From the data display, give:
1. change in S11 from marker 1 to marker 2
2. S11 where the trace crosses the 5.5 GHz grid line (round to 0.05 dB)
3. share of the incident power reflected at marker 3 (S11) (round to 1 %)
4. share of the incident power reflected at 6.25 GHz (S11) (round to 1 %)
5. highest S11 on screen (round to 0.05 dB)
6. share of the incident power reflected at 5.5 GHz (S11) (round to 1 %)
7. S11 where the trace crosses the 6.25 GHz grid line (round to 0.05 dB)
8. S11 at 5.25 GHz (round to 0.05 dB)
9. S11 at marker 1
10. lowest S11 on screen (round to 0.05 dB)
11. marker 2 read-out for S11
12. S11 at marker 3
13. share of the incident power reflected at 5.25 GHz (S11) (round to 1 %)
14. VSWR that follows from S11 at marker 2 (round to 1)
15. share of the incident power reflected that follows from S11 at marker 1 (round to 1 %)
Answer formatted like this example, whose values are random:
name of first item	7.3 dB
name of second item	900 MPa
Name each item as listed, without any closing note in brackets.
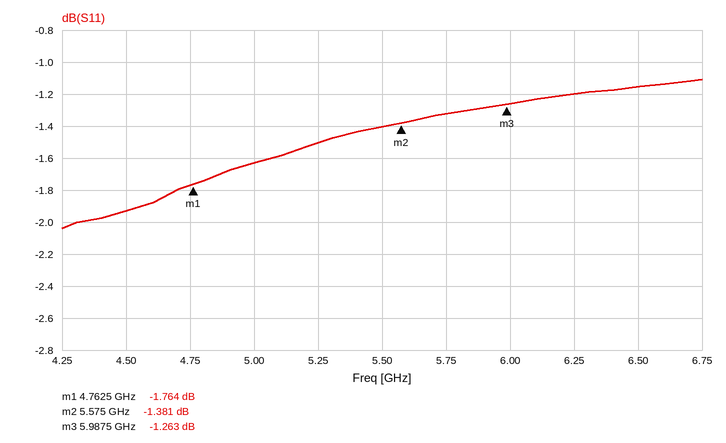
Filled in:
change in S11 from marker 1 to marker 2	0.383 dB
S11 where the trace crosses the 5.5 GHz grid line	-1.40 dB
share of the incident power reflected at marker 3 (S11)	75 %
share of the incident power reflected at 6.25 GHz (S11)	76 %
highest S11 on screen	-1.10 dB
share of the incident power reflected at 5.5 GHz (S11)	72 %
S11 where the trace crosses the 6.25 GHz grid line	-1.20 dB
S11 at 5.25 GHz	-1.50 dB
S11 at marker 1	-1.764 dB
lowest S11 on screen	-2.05 dB
marker 2 read-out for S11	-1.381 dB
S11 at marker 3	-1.263 dB
share of the incident power reflected at 5.25 GHz (S11)	71 %
VSWR that follows from S11 at marker 2	13
share of the incident power reflected that follows from S11 at marker 1	67 %
